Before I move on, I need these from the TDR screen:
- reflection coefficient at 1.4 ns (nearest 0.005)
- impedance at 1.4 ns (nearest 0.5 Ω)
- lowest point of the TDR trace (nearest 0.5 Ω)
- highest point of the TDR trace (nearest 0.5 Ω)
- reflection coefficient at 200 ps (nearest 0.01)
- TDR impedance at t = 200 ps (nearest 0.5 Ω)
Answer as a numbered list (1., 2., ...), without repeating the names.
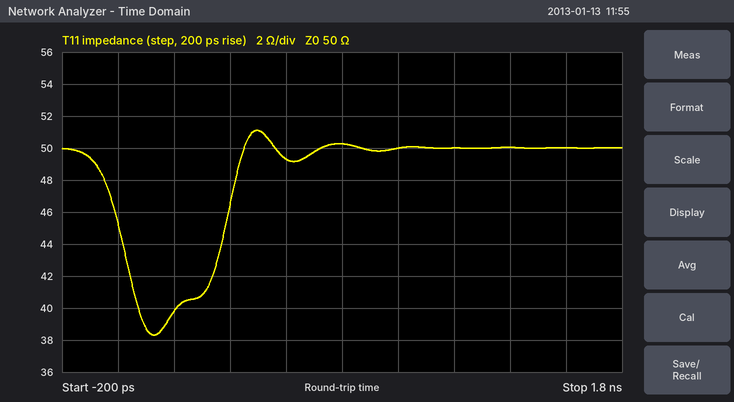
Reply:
1. 0.000
2. 50.0 Ω
3. 38.5 Ω
4. 51.0 Ω
5. -0.11
6. 40.0 Ω
